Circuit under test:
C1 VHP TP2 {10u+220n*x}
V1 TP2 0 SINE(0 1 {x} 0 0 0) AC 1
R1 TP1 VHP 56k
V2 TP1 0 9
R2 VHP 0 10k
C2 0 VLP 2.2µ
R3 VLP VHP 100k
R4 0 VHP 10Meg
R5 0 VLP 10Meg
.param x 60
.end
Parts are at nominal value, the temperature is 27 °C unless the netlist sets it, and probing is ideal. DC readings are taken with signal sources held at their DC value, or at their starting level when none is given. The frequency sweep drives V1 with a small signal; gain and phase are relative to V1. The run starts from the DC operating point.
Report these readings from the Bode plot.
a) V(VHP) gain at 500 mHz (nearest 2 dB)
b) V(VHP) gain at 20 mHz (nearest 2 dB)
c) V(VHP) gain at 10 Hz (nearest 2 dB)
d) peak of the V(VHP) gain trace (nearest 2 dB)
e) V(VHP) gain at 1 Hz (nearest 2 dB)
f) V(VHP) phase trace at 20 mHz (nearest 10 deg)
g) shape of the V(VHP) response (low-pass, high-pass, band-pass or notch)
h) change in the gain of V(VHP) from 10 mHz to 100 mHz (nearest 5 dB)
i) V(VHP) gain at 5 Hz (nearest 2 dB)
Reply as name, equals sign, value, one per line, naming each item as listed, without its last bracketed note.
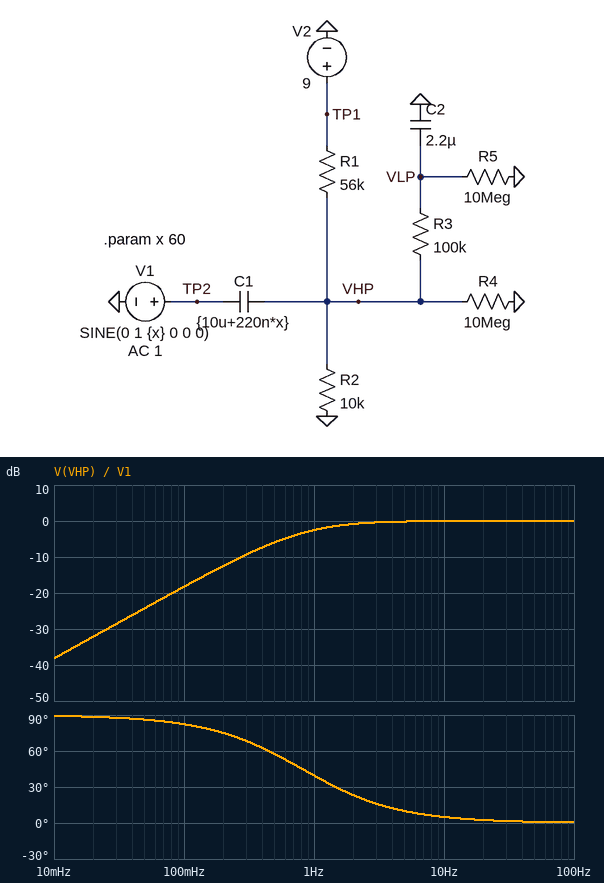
V(VHP) gain at 500 mHz = -6 dB
V(VHP) gain at 20 mHz = -32 dB
V(VHP) gain at 10 Hz = 0 dB
peak of the V(VHP) gain trace = 0 dB
V(VHP) gain at 1 Hz = -2 dB
V(VHP) phase trace at 20 mHz = 90 deg
shape of the V(VHP) response = high-pass
change in the gain of V(VHP) from 10 mHz to 100 mHz = 20 dB
V(VHP) gain at 5 Hz = 0 dB
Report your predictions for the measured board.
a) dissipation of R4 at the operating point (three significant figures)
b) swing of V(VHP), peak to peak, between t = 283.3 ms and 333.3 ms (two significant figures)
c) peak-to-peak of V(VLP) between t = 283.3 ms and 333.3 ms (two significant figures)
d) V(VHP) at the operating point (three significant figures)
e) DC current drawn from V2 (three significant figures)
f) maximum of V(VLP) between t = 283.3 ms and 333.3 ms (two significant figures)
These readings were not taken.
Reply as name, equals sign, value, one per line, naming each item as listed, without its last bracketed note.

dissipation of R4 at the operating point = 185 nW
swing of V(VHP), peak to peak, between t = 283.3 ms and 333.3 ms = 2.0 V
peak-to-peak of V(VLP) between t = 283.3 ms and 333.3 ms = 24 mV
V(VHP) at the operating point = 1.36 V
DC current drawn from V2 = 136 µA
maximum of V(VLP) between t = 283.3 ms and 333.3 ms = 1.4 V
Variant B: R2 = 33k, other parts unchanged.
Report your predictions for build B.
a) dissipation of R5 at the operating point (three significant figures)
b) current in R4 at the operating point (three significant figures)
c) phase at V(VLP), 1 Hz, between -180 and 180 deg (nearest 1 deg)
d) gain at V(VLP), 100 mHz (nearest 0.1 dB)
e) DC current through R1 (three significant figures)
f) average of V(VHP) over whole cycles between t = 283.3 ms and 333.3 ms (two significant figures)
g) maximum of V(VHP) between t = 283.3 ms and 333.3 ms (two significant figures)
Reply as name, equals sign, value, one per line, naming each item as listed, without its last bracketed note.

dissipation of R5 at the operating point = 1.08 µW
current in R4 at the operating point = 332 nA
phase at V(VLP), 1 Hz, between -180 and 180 deg = -34 deg
gain at V(VLP), 100 mHz = -11.1 dB
DC current through R1 = 101 µA
average of V(VHP) over whole cycles between t = 283.3 ms and 333.3 ms = 3.3 V
maximum of V(VHP) between t = 283.3 ms and 333.3 ms = 4.3 V
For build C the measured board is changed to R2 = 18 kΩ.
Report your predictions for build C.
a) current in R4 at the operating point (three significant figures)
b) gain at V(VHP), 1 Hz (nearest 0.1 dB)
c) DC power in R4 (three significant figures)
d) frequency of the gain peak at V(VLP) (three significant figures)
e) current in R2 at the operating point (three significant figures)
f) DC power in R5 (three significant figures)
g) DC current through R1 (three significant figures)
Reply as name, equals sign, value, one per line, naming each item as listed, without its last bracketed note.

current in R4 at the operating point = 218 nA
gain at V(VHP), 1 Hz = -1.4 dB
DC power in R4 = 477 nW
frequency of the gain peak at V(VLP) = 607 mHz
current in R2 at the operating point = 121 µA
DC power in R5 = 467 nW
DC current through R1 = 122 µA
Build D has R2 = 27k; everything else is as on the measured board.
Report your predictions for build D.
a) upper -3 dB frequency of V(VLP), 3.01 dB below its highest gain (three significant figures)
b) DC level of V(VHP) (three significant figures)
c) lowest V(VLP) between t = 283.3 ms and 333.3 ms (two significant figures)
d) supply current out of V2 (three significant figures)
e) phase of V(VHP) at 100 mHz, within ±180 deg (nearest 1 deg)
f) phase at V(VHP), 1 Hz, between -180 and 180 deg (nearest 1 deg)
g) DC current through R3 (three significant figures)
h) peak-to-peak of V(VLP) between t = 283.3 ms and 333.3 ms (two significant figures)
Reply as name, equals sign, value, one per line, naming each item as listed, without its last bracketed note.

upper -3 dB frequency of V(VLP), 3.01 dB below its highest gain = 1.38 Hz
DC level of V(VHP) = 2.92 V
lowest V(VLP) between t = 283.3 ms and 333.3 ms = 2.9 V
supply current out of V2 = 109 µA
phase of V(VHP) at 100 mHz, within ±180 deg = 74 deg
phase at V(VHP), 1 Hz, between -180 and 180 deg = 22 deg
DC current through R3 = 289 nA
peak-to-peak of V(VLP) between t = 283.3 ms and 333.3 ms = 25 mV
